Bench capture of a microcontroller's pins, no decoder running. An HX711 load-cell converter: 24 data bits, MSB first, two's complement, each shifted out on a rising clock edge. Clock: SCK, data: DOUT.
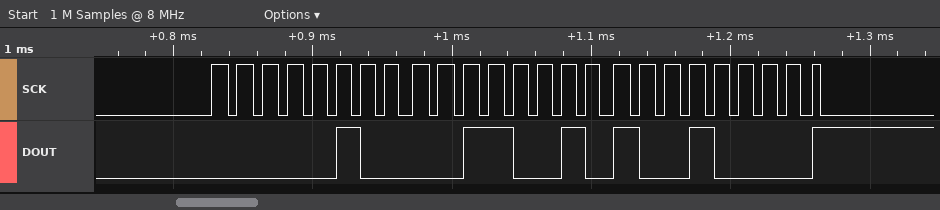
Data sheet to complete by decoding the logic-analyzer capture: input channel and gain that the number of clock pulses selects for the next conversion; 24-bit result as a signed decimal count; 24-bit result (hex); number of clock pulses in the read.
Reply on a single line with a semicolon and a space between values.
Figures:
channel A, gain 128; 275088; 0x043290; 25
